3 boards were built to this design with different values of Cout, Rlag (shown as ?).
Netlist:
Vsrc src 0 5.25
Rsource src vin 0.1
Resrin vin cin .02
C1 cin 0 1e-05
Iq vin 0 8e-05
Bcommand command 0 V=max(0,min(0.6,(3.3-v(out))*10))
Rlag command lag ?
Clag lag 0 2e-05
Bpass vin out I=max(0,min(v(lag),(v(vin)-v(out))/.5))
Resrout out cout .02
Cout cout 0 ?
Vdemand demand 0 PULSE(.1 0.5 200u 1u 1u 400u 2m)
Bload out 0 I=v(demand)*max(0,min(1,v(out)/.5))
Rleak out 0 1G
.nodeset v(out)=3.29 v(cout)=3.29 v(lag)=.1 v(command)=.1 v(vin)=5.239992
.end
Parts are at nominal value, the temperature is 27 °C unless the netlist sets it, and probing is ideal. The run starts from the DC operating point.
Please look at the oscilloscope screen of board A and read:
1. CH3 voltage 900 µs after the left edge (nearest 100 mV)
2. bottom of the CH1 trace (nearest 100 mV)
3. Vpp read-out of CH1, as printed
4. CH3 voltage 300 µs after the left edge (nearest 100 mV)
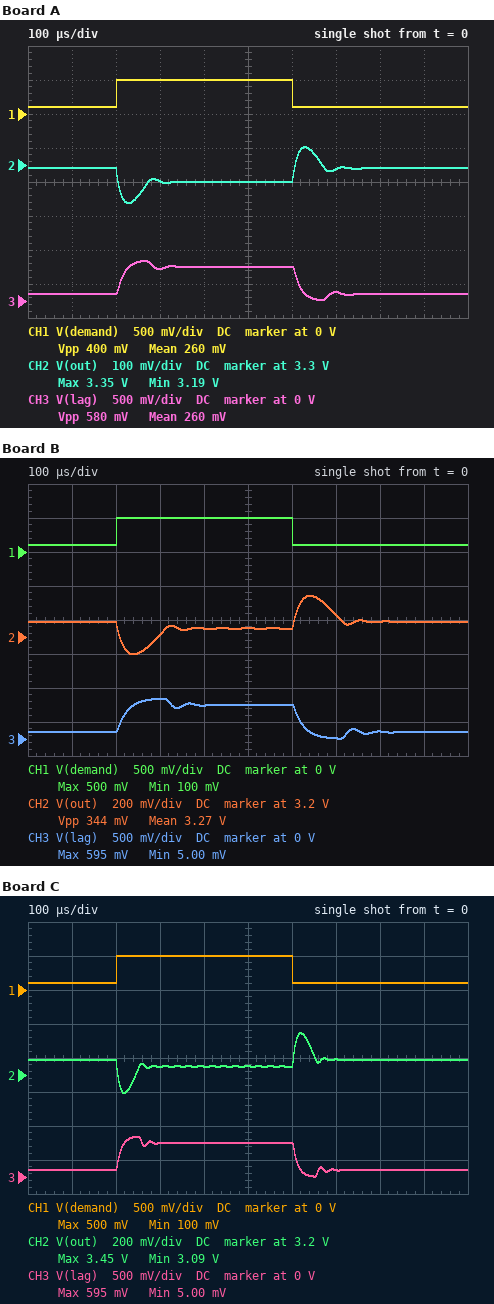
100 mV
100 mV
400 mV
500 mV
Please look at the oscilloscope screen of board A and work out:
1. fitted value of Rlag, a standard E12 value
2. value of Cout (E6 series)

0.82 Ω
47 µF
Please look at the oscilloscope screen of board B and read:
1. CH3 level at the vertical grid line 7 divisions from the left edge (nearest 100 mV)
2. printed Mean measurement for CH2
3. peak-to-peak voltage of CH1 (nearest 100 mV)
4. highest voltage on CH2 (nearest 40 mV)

0 V
3.27 V
400 mV
3.44 V
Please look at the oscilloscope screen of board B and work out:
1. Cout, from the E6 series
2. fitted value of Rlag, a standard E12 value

33 µF
1.2 Ω
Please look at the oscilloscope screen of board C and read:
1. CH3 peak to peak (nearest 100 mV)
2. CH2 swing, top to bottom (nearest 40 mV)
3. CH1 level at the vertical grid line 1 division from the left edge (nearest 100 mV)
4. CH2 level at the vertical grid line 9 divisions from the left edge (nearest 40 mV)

600 mV
360 mV
100 mV
3.28 V
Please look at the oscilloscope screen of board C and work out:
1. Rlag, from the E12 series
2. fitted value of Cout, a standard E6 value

0.56 Ω
15 µF
